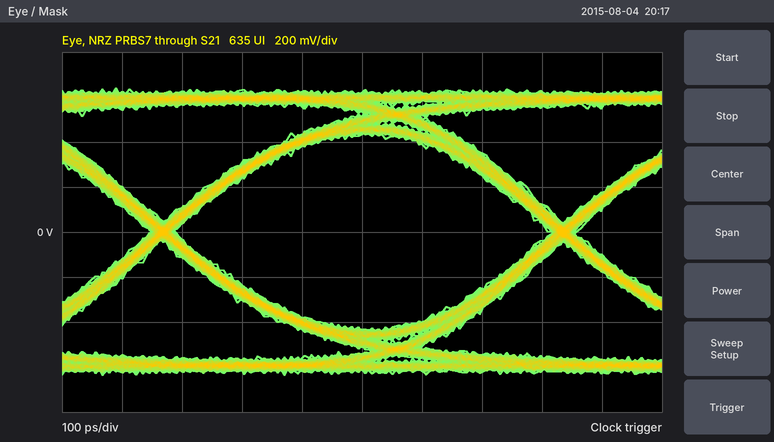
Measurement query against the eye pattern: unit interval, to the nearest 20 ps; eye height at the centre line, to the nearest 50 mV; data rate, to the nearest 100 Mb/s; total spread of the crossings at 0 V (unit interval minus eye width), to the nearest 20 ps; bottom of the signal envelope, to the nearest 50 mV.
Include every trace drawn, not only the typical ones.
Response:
660 ps
850 mV
1.5 Gb/s
40 ps
-650 mV
